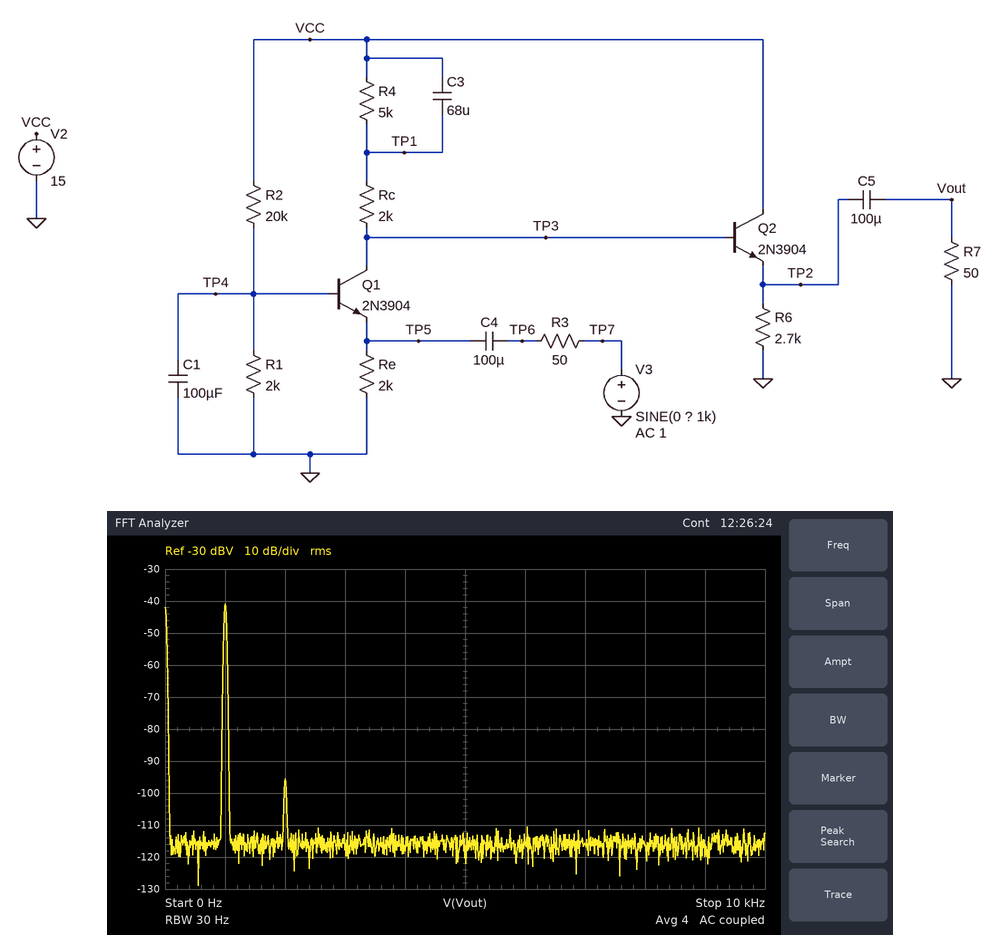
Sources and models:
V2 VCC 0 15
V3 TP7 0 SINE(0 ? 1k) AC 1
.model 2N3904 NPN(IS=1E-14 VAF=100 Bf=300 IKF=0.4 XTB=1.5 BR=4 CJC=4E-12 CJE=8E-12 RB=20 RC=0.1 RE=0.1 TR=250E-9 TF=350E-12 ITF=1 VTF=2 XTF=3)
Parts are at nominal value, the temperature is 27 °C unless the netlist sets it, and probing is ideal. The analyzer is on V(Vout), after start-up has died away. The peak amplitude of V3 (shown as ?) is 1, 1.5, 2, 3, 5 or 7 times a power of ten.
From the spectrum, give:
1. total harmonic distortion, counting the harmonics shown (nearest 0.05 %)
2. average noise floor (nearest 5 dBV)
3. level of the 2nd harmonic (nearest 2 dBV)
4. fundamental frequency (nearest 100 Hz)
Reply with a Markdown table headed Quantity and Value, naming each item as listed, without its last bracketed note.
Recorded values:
| Quantity | Value |
|---|---|
| total harmonic distortion, counting the harmonics shown | 0.20 % |
| average noise floor | -115 dBV |
| level of the 2nd harmonic | -96 dBV |
| fundamental frequency | 1.0 kHz |
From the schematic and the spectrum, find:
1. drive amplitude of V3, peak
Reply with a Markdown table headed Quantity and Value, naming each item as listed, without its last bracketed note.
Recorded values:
| Quantity | Value |
|---|---|
| drive amplitude of V3, peak | 1 mV |
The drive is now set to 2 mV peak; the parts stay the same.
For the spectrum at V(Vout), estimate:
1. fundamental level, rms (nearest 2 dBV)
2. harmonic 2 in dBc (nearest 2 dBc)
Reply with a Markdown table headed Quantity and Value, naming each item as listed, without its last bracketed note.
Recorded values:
| Quantity | Value |
|---|---|
| fundamental level, rms | -34 dBV |
| harmonic 2 in dBc | -48 dBc |
